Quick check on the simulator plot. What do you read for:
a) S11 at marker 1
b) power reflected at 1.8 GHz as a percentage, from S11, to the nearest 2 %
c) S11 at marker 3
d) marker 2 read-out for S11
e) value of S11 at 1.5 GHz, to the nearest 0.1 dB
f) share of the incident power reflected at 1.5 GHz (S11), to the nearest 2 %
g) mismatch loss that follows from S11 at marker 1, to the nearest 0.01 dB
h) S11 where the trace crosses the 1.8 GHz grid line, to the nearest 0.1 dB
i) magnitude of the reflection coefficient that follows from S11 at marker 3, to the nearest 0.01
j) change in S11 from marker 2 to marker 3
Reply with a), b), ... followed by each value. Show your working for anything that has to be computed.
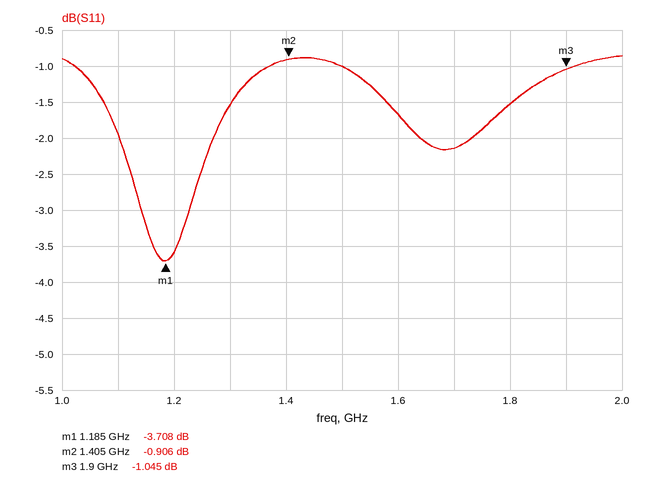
a) -3.708 dB
b) 10^(-1.5/10) ≈ 70.8 %, so 70 % to the nearest 2 %
c) -1.045 dB
d) -0.906 dB
e) -1.0 dB
f) 10^(-1/10) ≈ 79.4 %, so 80 % to the nearest 2 %
g) −10 log10(1 − 10^(-3.708/10)) ≈ 2.41 dB
h) -1.5 dB
i) 10^(-1.045/20) ≈ 0.89
j) -1.045 − (-0.906) = -0.139 dB
